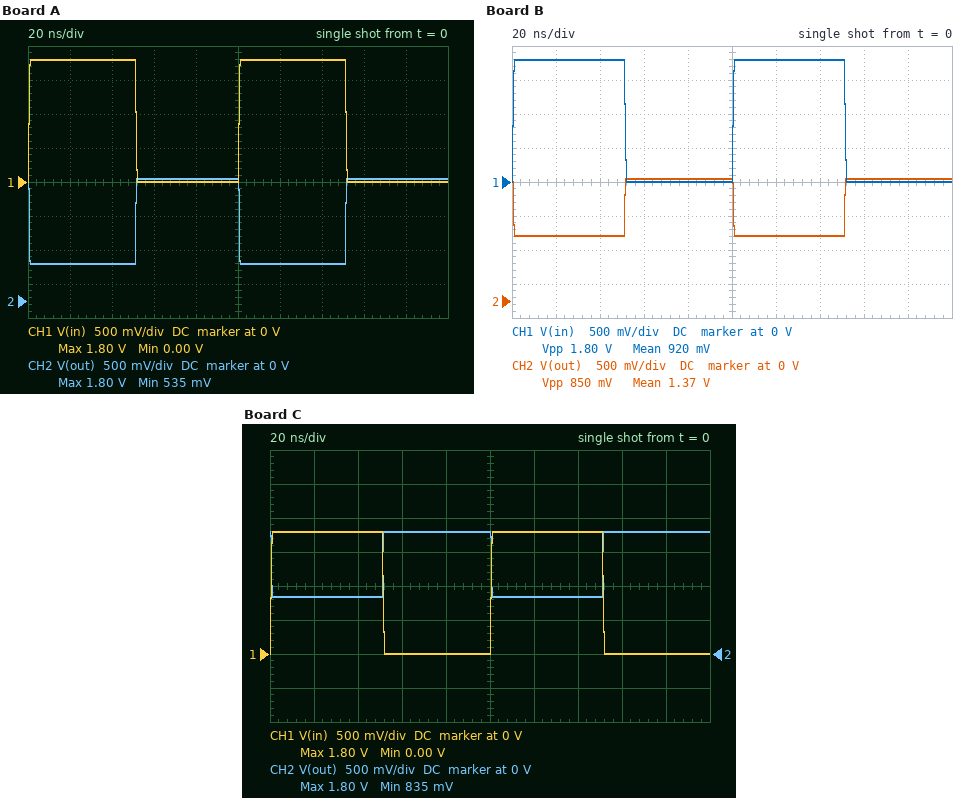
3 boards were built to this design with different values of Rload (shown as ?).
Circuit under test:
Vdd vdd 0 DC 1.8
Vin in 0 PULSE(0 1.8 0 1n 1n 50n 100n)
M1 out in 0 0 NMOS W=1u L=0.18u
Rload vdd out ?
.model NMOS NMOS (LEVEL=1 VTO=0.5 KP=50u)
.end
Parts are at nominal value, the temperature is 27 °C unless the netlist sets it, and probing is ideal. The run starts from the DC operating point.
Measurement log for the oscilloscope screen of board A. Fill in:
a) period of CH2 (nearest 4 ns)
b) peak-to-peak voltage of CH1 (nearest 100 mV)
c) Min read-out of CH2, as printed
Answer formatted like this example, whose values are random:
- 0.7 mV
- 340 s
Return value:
- 100 ns
- 1.8 V
- 535 mV
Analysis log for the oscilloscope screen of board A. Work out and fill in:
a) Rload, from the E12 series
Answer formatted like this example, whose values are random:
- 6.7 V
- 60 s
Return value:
- 8.2 kΩ
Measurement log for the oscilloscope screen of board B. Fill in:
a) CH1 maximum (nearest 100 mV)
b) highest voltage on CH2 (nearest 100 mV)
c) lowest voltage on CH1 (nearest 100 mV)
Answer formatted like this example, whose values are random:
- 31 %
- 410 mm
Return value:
- 1.8 V
- 1.8 V
- 0 V
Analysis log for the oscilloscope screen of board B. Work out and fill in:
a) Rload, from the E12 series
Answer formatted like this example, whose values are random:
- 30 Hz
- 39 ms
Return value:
- 3.9 kΩ
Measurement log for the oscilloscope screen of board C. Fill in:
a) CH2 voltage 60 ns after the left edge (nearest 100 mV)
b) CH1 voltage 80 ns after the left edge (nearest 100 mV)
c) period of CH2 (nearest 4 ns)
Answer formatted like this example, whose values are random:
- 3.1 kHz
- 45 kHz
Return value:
- 1.8 V
- 0 V
- 100 ns
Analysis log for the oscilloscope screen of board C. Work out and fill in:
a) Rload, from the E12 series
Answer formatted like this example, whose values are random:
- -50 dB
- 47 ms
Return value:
- 4.7 kΩ
